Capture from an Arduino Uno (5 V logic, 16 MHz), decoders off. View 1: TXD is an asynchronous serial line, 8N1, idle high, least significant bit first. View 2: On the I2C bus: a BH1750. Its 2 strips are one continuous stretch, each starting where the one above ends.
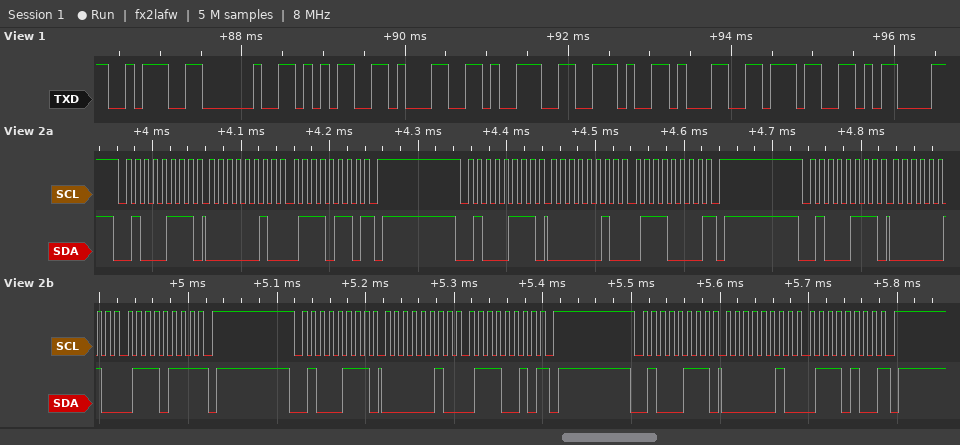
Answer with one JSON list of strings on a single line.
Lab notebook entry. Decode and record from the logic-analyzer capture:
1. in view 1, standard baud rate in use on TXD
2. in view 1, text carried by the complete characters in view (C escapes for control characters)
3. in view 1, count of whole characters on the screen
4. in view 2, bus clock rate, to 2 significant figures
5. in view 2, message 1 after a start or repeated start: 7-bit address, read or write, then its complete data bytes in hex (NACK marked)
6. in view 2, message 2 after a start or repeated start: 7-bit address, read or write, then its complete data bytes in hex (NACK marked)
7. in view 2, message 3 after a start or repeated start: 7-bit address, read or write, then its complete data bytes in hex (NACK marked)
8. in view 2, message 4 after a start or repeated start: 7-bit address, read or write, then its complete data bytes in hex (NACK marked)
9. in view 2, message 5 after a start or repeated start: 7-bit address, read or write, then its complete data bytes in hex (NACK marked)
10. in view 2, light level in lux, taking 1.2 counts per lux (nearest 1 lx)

["9600 baud", "\": 519.17\\r\"", "9", "100 kHz", "0x23 read: 02 76 NACK", "0x23 read: 02 70 NACK", "0x23 read: 02 77 NACK", "0x23 read: 02 72 NACK", "0x23 read: 02 74 NACK", "525 lx"]
